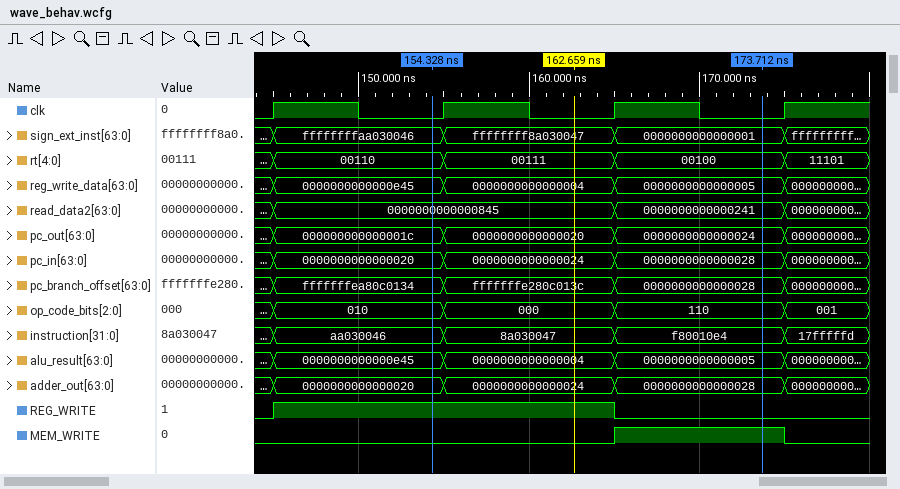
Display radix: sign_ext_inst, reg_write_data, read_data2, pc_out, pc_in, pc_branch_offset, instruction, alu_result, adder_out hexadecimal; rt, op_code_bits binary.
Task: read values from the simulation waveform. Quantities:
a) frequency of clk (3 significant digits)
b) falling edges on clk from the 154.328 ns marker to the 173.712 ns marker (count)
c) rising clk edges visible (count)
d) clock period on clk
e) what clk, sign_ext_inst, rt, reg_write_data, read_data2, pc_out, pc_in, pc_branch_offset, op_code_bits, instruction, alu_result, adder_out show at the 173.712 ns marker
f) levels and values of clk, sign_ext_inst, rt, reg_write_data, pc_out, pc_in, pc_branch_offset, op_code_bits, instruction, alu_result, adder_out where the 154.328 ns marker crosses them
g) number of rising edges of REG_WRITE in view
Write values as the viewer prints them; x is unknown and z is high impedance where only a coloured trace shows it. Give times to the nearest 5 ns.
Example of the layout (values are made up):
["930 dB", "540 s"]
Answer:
["100 MHz", "2", "4", "10 ns", "clk=0, sign_ext_inst=0000000000000001, rt=00100, reg_write_data=0000000000000005, read_data2=0000000000000241, pc_out=0000000000000024, pc_in=0000000000000028, pc_branch_offset=0000000000000028, op_code_bits=110, instruction=f80010e4, alu_result=0000000000000005, adder_out=0000000000000028", "clk=0, sign_ext_inst=ffffffffaa030046, rt=00110, reg_write_data=0000000000000e45, pc_out=000000000000001c, pc_in=0000000000000020, pc_branch_offset=fffffffea80c0134, op_code_bits=010, instruction=aa030046, alu_result=0000000000000e45, adder_out=0000000000000020", "1"]
